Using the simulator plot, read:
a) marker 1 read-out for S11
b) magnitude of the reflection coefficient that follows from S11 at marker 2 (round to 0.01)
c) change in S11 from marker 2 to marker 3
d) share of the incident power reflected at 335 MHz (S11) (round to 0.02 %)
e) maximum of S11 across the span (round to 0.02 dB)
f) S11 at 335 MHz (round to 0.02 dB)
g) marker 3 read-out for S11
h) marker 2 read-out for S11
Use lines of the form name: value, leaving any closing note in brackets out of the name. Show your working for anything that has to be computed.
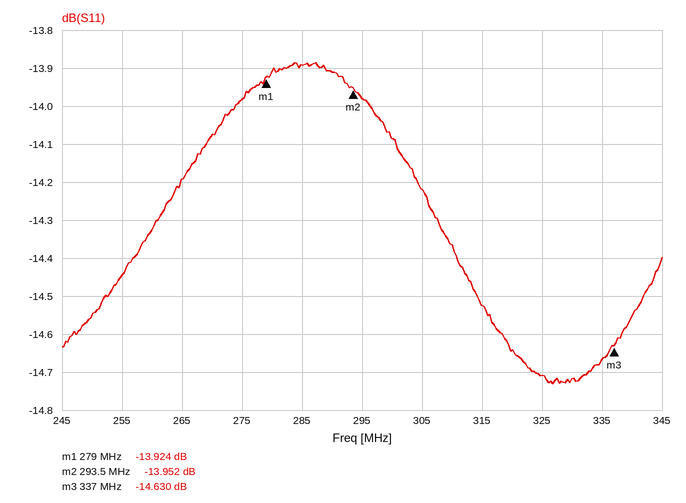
marker 1 read-out for S11: -13.924 dB
magnitude of the reflection coefficient that follows from S11 at marker 2: 10^(-13.952/20) ≈ 0.20
change in S11 from marker 2 to marker 3: -14.63 − (-13.952) = -0.678 dB
share of the incident power reflected at 335 MHz (S11): 10^(-14.66/10) ≈ 3.42 %
maximum of S11 across the span: -13.88 dB
S11 at 335 MHz: -14.66 dB
marker 3 read-out for S11: -14.630 dB
marker 2 read-out for S11: -13.952 dB
